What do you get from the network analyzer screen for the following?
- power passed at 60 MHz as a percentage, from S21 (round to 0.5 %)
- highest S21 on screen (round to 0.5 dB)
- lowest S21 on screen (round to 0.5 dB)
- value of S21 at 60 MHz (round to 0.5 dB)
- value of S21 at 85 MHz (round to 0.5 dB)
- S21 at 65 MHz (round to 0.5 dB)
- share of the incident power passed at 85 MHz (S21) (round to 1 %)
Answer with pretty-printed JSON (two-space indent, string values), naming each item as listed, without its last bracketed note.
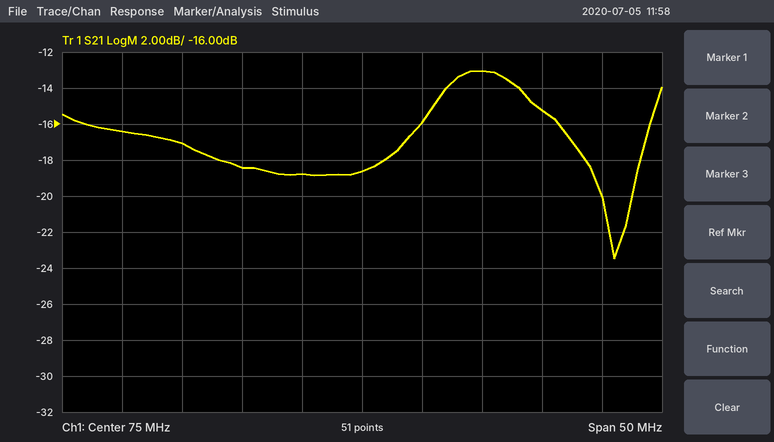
{
  "power passed at 60 MHz as a percentage, from S21": "2.0 %",
  "highest S21 on screen": "-13.0 dB",
  "lowest S21 on screen": "-23.5 dB",
  "value of S21 at 60 MHz": "-17.0 dB",
  "value of S21 at 85 MHz": "-13.0 dB",
  "S21 at 65 MHz": "-18.5 dB",
  "share of the incident power passed at 85 MHz (S21)": "5 %"
}
